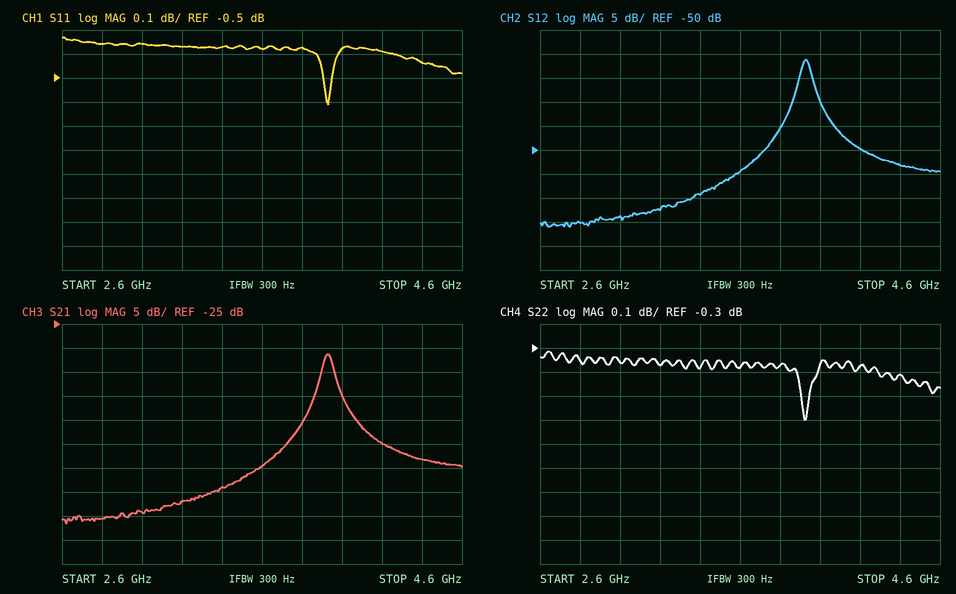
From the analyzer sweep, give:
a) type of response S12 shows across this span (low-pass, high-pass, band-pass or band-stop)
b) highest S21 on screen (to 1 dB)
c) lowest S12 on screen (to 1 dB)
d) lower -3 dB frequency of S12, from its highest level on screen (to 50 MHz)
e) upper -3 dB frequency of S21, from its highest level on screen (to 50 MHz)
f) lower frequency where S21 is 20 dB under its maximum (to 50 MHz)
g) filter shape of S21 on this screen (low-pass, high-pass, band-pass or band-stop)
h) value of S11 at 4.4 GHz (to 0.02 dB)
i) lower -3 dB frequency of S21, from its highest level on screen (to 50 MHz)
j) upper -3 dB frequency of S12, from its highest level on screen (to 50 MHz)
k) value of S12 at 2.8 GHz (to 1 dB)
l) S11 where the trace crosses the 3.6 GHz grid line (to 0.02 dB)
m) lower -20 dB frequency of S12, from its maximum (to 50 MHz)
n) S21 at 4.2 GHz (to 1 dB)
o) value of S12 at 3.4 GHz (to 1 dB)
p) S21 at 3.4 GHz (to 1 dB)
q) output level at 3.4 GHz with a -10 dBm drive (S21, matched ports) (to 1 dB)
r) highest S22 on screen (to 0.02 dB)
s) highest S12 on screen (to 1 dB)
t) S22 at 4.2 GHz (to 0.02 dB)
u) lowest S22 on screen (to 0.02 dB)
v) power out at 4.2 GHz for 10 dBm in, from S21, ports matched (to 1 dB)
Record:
band-pass
-31 dB
-66 dB
3.90 GHz
3.95 GHz
3.70 GHz
band-pass
-0.44 dB
3.90 GHz
3.95 GHz
-65 dB
-0.38 dB
3.70 GHz
-50 dB
-59 dB
-59 dB
-69 dBm
-0.32 dB
-31 dB
-0.38 dB
-0.60 dB
-40 dBm
